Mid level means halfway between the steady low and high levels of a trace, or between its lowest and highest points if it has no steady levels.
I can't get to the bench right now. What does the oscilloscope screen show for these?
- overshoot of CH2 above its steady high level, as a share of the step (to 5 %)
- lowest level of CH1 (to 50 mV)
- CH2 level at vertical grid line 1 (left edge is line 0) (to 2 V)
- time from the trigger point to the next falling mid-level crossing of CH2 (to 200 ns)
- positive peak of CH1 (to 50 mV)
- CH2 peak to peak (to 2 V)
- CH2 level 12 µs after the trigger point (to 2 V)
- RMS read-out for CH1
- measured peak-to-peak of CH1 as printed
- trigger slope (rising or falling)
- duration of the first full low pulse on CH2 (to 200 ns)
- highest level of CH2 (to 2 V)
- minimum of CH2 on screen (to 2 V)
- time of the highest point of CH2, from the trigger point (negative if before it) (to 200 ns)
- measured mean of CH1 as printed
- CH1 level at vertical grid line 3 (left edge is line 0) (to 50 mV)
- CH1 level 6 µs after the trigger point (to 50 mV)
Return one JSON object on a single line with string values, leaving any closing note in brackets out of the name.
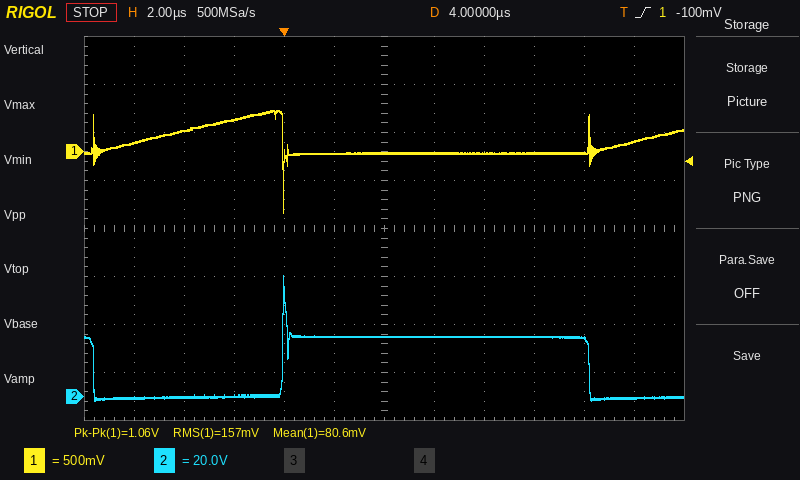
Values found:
{"overshoot of CH2 above its steady high level, as a share of the step": "100 %", "lowest level of CH1": "-650 mV", "CH2 level at vertical grid line 1 (left edge is line 0)": "0 V", "time from the trigger point to the next falling mid-level crossing of CH2": "12.2 µs", "positive peak of CH1": "450 mV", "CH2 peak to peak": "52 V", "CH2 level 12 µs after the trigger point": "24 V", "RMS read-out for CH1": "157 mV", "measured peak-to-peak of CH1 as printed": "1.06 V", "trigger slope": "rising", "duration of the first full low pulse on CH2": "7.6 µs", "highest level of CH2": "50 V", "minimum of CH2 on screen": "-2 V", "time of the highest point of CH2, from the trigger point (negative if before it)": "0.0 µs", "measured mean of CH1 as printed": "80.6 mV", "CH1 level at vertical grid line 3 (left edge is line 0)": "350 mV", "CH1 level 6 µs after the trigger point": "0 mV"}
